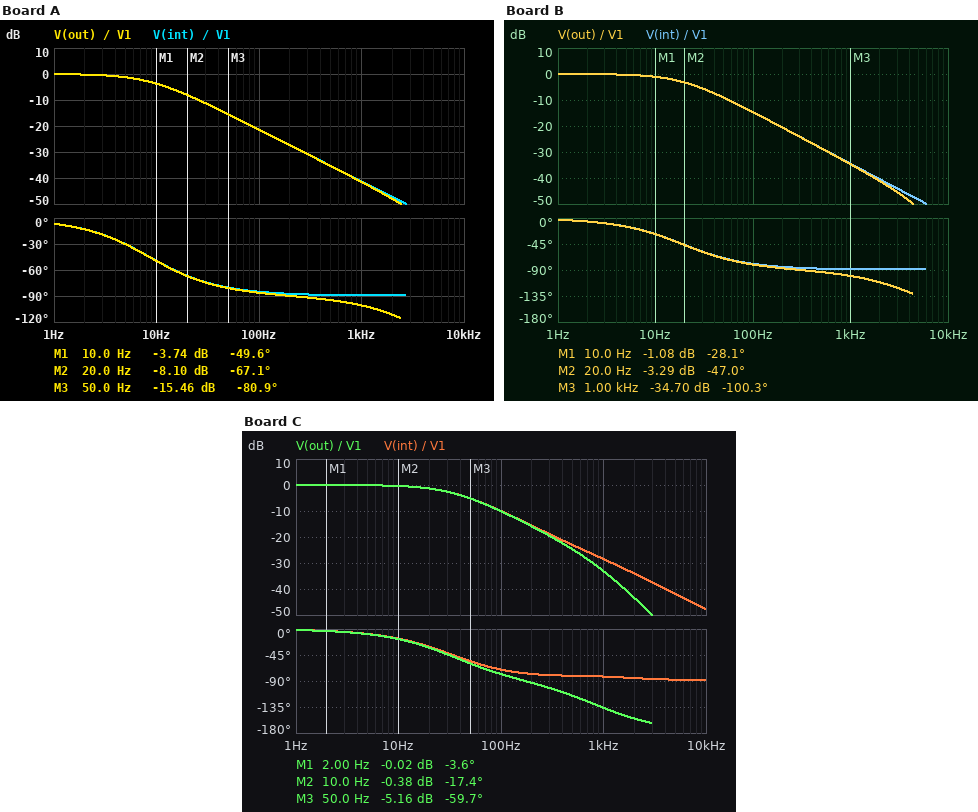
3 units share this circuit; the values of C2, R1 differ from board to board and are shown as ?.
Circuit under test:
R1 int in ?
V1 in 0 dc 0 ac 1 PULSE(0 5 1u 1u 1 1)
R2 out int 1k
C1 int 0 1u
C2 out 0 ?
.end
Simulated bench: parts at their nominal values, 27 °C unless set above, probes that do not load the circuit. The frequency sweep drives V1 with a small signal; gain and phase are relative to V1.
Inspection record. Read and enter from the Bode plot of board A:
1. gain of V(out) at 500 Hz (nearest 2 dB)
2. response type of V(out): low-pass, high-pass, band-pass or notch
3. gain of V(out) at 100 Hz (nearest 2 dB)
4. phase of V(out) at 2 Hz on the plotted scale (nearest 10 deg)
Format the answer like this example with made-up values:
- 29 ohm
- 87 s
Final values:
- -36 dB
- low-pass
- -22 dB
- -10 deg
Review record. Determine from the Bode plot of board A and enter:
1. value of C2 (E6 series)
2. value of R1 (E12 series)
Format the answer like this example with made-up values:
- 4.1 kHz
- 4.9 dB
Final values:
- 33 nF
- 18 kΩ
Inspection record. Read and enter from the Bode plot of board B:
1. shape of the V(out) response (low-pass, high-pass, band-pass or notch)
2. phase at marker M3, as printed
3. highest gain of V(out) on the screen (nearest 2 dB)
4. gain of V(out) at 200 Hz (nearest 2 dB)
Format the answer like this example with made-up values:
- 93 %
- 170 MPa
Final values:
- low-pass
- -100.3 deg
- 0 dB
- -20 dB
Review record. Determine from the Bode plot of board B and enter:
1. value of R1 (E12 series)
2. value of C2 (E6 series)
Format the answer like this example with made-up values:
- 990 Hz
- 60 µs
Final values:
- 8.2 kΩ
- 33 nF
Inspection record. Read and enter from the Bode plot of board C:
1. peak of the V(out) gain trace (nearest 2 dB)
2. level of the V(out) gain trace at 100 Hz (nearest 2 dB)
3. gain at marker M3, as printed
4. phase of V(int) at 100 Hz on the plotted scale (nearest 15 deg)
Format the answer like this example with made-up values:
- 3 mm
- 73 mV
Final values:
- 0 dB
- -10 dB
- -5.16 dB
- -75 deg
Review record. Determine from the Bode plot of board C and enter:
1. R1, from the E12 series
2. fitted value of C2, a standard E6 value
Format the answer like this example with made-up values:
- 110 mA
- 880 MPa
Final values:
- 3.9 kΩ
- 220 nF
